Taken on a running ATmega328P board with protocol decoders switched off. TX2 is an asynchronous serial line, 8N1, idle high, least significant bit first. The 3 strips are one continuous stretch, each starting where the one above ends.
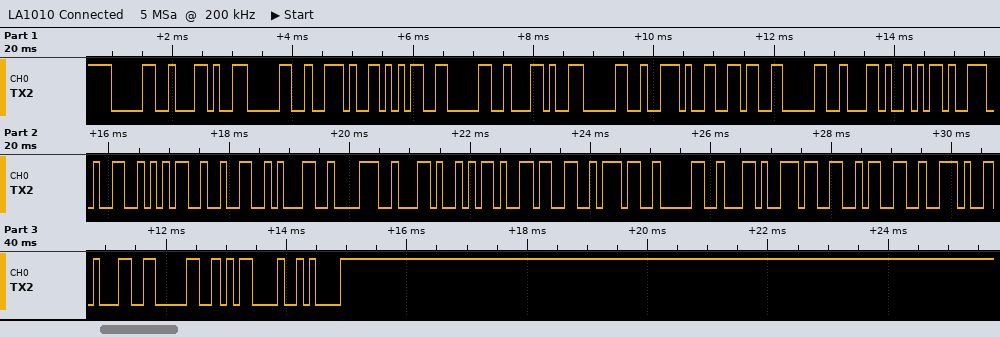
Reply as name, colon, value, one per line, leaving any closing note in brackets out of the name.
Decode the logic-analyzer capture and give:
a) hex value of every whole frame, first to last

hex value of every whole frame, first to last: 30 2C 30 2E 35 30 2C 30 2E 36 30 2C 2D 32 35 32 31 38 2C 2D 33 37 30 2C 33 33 2E 31 30 0D 0A
